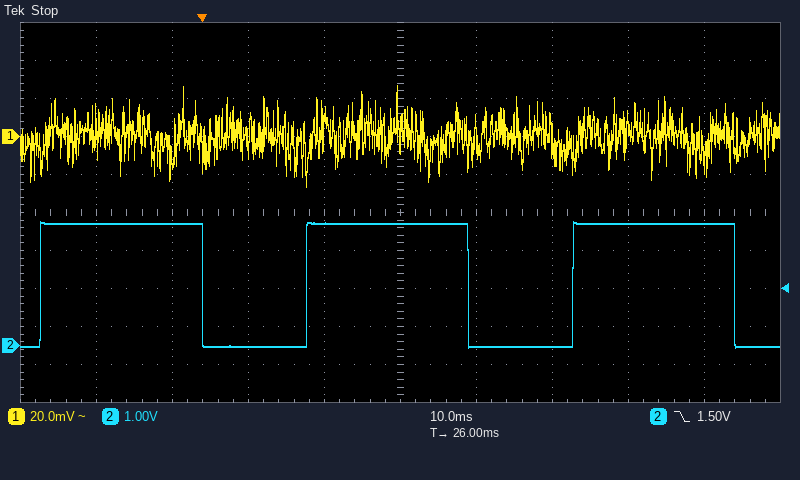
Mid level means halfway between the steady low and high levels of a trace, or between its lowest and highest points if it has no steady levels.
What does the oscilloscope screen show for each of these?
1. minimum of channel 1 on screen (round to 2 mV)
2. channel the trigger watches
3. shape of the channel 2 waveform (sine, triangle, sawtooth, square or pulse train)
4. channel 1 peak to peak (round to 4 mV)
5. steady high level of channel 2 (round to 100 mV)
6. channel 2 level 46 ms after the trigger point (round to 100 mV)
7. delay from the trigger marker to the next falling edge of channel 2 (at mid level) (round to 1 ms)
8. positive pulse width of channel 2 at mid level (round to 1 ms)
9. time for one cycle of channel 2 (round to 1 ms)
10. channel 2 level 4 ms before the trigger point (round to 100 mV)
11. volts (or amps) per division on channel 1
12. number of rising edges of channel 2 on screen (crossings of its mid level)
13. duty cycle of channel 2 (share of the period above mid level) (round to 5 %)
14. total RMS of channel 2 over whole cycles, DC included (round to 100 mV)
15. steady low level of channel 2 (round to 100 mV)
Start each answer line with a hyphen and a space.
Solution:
- -26 mV
- channel 2
- pulse train
- 52 mV
- 3.2 V
- 0.0 V
- 35 ms
- 21 ms
- 35 ms
- 3.2 V
- 20 mV
- 3
- 60 %
- 2.5 V
- 0.0 V
